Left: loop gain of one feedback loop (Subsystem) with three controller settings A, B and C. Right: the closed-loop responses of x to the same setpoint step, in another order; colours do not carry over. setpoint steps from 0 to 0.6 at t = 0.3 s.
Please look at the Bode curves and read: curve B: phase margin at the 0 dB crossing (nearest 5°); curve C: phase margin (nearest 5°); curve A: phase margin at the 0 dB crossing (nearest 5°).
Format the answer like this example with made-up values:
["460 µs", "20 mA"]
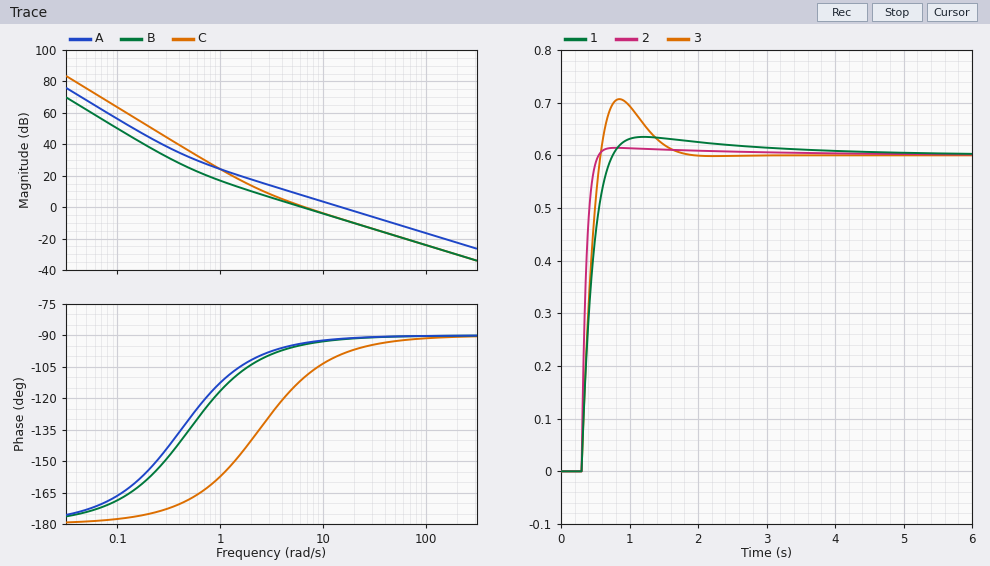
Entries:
["85°", "70°", "90°"]
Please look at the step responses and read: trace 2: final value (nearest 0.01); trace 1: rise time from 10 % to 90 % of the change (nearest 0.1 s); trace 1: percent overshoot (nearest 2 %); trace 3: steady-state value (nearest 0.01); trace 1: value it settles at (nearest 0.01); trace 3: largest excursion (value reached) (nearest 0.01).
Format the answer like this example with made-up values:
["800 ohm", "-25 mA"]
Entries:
["0.60", "0.3 s", "6 %", "0.60", "0.60", "0.71"]
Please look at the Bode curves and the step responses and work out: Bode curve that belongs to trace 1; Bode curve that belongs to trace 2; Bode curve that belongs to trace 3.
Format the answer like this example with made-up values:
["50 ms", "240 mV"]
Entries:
["B", "A", "C"]
